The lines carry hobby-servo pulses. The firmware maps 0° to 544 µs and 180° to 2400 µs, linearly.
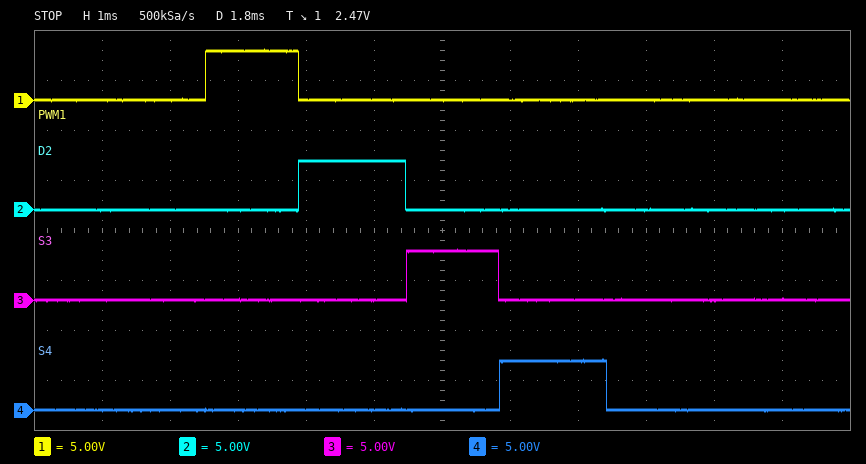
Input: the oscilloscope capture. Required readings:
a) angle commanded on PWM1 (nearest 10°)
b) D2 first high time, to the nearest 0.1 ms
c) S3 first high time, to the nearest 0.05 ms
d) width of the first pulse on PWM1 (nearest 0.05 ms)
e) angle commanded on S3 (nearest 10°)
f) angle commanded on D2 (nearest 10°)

80°
1.6 ms
1.35 ms
1.35 ms
80°
100°
